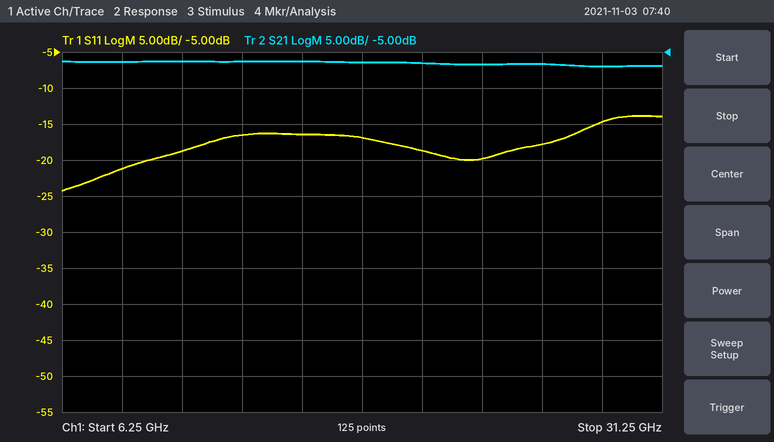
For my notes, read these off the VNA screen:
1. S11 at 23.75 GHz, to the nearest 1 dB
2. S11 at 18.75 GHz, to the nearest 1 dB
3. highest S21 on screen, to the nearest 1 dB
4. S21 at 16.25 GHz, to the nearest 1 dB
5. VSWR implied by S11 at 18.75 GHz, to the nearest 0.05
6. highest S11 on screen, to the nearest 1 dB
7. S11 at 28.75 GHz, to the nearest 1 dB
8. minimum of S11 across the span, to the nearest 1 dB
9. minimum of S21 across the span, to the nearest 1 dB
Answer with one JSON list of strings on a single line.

["-20 dB", "-17 dB", "-6 dB", "-6 dB", "1.35", "-14 dB", "-15 dB", "-24 dB", "-7 dB"]
